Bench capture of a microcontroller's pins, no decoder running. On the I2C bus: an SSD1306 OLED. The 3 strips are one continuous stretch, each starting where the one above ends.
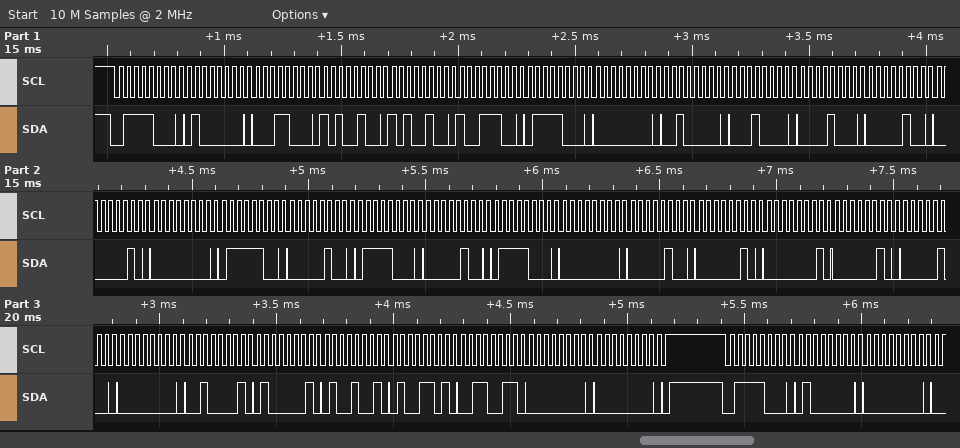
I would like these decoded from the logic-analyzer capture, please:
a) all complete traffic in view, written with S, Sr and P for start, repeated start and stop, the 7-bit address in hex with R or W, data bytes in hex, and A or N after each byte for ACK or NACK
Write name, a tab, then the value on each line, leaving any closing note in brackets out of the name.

all complete traffic in view, written with S, Sr and P for start, repeated start and stop, the 7-bit address in hex with R or W, data bytes in hex, and A or N after each byte for ACK or NACK	S 3CW A 40 A 18 A A4 A A4 A 9C A 78 A 00 A 20 A 10 A 08 A 04 A 02 A 00 A 7C A 04 A 78 A 04 A 78 A 00 A 04 A 02 A 01 A 02 A 04 A 00 A 21 A 41 A 49 A 4D A 33 A 00 A 00 A P S 3CW A 40 A 00 A
